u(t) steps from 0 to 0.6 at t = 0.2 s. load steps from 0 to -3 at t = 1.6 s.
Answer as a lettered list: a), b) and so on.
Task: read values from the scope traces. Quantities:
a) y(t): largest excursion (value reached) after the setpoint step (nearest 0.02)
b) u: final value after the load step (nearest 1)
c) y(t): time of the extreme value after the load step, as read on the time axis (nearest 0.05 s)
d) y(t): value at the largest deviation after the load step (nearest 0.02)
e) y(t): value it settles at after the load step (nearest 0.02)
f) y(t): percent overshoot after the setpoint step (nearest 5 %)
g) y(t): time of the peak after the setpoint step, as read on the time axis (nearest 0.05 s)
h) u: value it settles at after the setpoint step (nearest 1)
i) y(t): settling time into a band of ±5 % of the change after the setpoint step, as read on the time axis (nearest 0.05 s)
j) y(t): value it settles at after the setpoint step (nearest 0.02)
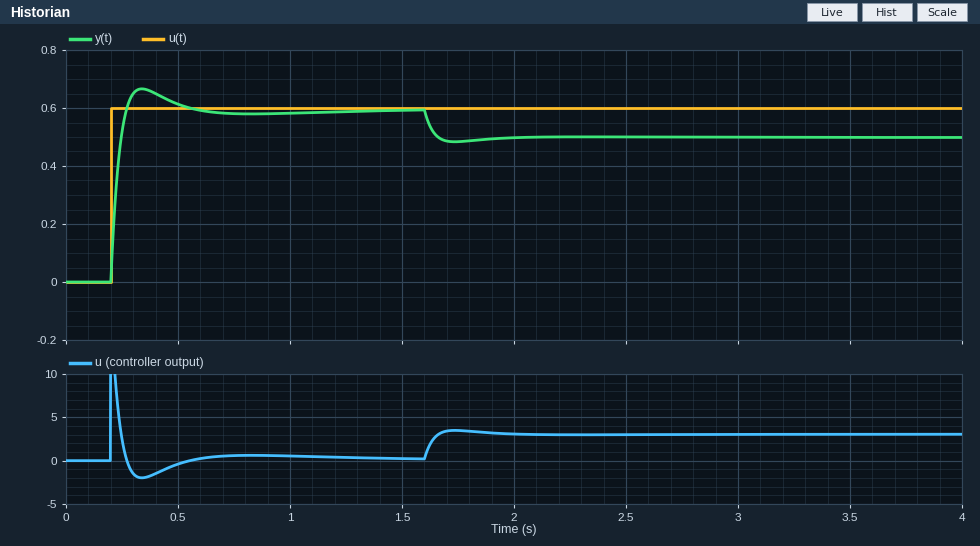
a) 0.66
b) 3
c) 1.75 s
d) 0.48
e) 0.50
f) 10 %
g) 0.35 s
h) 0
i) 0.45 s
j) 0.60
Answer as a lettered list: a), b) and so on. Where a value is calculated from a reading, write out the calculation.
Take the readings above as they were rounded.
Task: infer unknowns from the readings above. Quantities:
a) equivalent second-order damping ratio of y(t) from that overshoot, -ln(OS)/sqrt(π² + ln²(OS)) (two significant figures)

a) ln(0.1) = -2.303; 2.303 / sqrt(9.870 + 5.302) = 0.59
